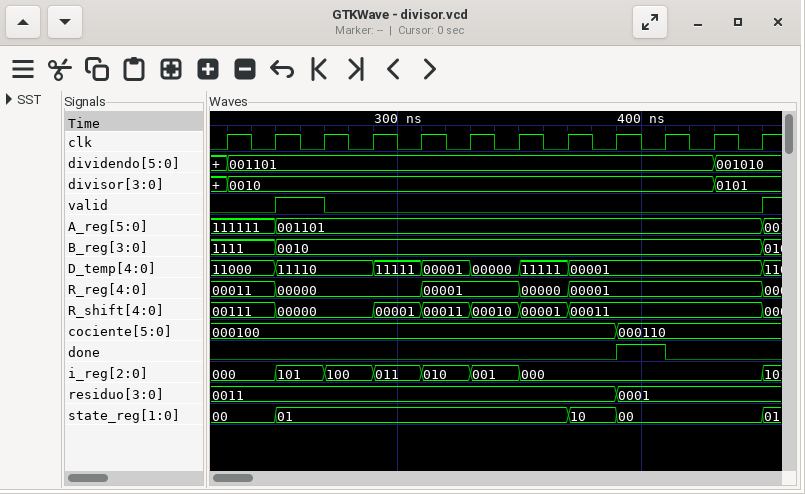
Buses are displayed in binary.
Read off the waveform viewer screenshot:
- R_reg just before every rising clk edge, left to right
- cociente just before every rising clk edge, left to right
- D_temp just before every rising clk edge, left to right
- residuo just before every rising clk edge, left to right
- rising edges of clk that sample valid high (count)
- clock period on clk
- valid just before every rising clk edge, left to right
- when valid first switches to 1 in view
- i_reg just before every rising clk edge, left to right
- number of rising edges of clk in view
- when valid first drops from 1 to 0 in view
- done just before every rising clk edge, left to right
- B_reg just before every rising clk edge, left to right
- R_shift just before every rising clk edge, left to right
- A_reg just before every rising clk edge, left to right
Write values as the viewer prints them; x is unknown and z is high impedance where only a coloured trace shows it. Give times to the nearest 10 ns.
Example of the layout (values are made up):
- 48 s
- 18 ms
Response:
- 00011, 00011, 00000, 00000, 00000, 00001, 00001, 00000, 00001, 00001, 00001, 00001
- 000100, 000100, 000100, 000100, 000100, 000100, 000100, 000100, 000100, 000110, 000110, 000110
- 11000, 11000, 11110, 11110, 11111, 00001, 00000, 11111, 00001, 00001, 00001, 00001
- 0011, 0011, 0011, 0011, 0011, 0011, 0011, 0011, 0011, 0001, 0001, 0001
- 1
- 20 ns
- 0 0 1 0 0 0 0 0 0 0 0 0
- 250 ns
- 000, 000, 101, 100, 011, 010, 001, 000, 000, 000, 000, 000
- 12
- 270 ns
- 0 0 0 0 0 0 0 0 0 1 0 0
- 1111, 1111, 0010, 0010, 0010, 0010, 0010, 0010, 0010, 0010, 0010, 0010
- 00111, 00111, 00000, 00000, 00001, 00011, 00010, 00001, 00011, 00011, 00011, 00011
- 111111, 111111, 001101, 001101, 001101, 001101, 001101, 001101, 001101, 001101, 001101, 001101
